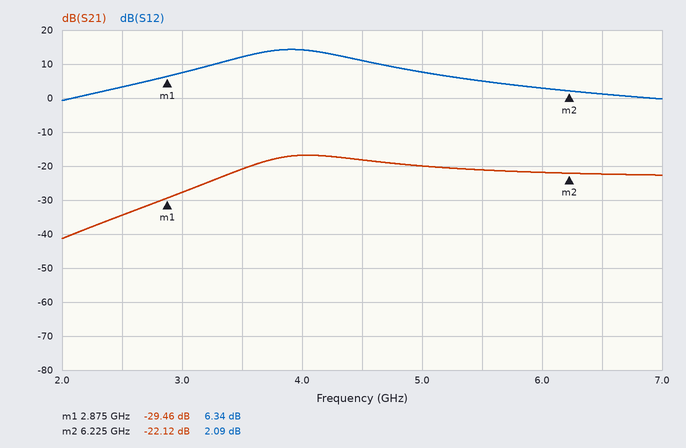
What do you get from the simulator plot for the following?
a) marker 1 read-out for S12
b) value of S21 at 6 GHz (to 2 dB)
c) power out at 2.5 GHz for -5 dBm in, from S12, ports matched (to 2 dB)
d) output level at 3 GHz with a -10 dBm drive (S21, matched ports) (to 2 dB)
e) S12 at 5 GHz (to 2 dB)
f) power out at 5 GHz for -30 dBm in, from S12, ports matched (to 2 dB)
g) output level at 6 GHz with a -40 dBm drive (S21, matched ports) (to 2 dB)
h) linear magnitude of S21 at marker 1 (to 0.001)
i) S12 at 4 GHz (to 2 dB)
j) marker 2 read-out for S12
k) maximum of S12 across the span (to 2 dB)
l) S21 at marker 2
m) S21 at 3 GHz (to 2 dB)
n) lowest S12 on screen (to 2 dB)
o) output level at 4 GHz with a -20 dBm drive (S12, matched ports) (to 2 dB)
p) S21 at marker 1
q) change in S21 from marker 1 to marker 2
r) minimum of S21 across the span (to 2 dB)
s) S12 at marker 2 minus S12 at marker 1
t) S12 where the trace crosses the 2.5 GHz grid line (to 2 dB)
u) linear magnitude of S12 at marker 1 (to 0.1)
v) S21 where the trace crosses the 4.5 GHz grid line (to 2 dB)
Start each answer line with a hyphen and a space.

- 6.34 dB
- -22 dB
- -2 dBm
- -38 dBm
- 8 dB
- -22 dBm
- -62 dBm
- 0.034
- 14 dB
- 2.09 dB
- 14 dB
- -22.12 dB
- -28 dB
- 0 dB
- -6 dBm
- -29.46 dB
- 7.34 dB
- -42 dB
- -4.25 dB
- 4 dB
- 2.1
- -18 dB
